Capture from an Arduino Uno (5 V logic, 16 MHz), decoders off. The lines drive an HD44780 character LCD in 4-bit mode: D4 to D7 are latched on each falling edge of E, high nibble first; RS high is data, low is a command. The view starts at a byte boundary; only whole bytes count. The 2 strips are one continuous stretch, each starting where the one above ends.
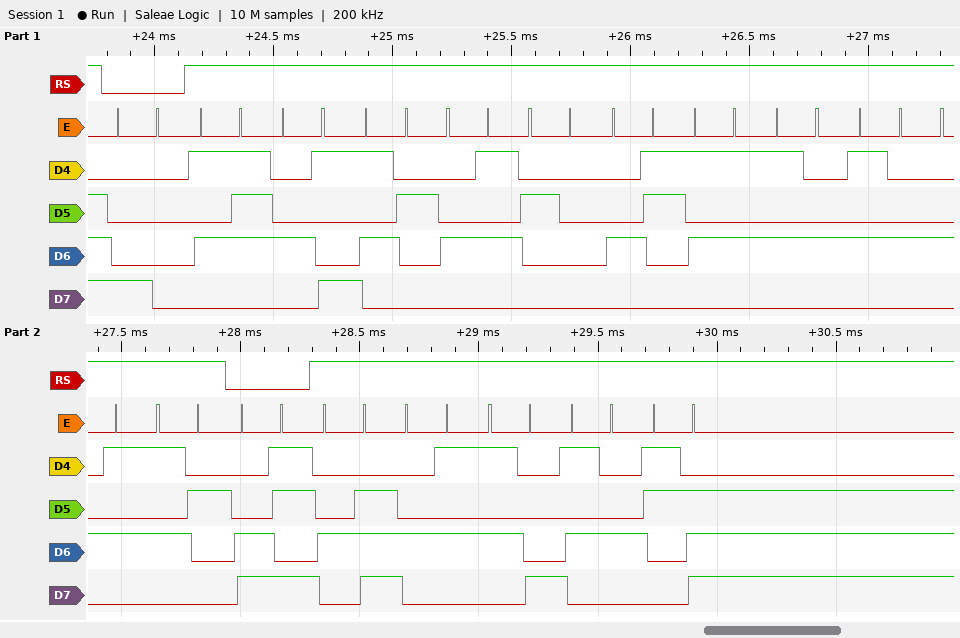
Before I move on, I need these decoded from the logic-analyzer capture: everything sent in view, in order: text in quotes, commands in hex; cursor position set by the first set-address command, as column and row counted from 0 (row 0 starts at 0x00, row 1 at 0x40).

0x80 "WIRE CUTTER" 0xCB "NEXT>"
column 0, row 0
